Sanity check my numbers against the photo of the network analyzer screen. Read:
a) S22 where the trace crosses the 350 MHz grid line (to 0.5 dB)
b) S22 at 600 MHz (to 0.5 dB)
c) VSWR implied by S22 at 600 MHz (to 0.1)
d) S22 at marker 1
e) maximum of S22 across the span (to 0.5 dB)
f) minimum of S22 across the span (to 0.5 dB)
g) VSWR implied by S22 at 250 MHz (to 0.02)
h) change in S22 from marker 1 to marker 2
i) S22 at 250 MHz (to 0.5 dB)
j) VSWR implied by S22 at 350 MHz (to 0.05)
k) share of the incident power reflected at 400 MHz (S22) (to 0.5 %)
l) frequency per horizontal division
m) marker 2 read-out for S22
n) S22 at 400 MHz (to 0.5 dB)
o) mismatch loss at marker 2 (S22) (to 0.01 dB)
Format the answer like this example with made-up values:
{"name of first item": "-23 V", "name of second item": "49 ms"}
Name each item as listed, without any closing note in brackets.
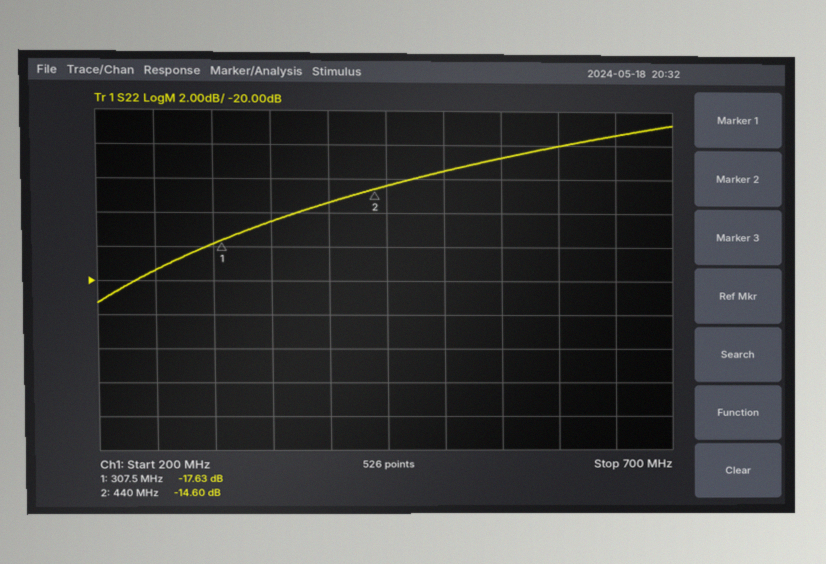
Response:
{"S22 where the trace crosses the 350 MHz grid line": "-16.5 dB", "S22 at 600 MHz": "-12.0 dB", "VSWR implied by S22 at 600 MHz": "1.7", "S22 at marker 1": "-17.63 dB", "maximum of S22 across the span": "-11.0 dB", "minimum of S22 across the span": "-21.5 dB", "VSWR implied by S22 at 250 MHz": "1.24", "change in S22 from marker 1 to marker 2": "3.03 dB", "S22 at 250 MHz": "-19.5 dB", "VSWR implied by S22 at 350 MHz": "1.35", "share of the incident power reflected at 400 MHz (S22)": "3.0 %", "frequency per horizontal division": "50 MHz", "marker 2 read-out for S22": "-14.60 dB", "S22 at 400 MHz": "-15.5 dB", "mismatch loss at marker 2 (S22)": "0.15 dB"}
